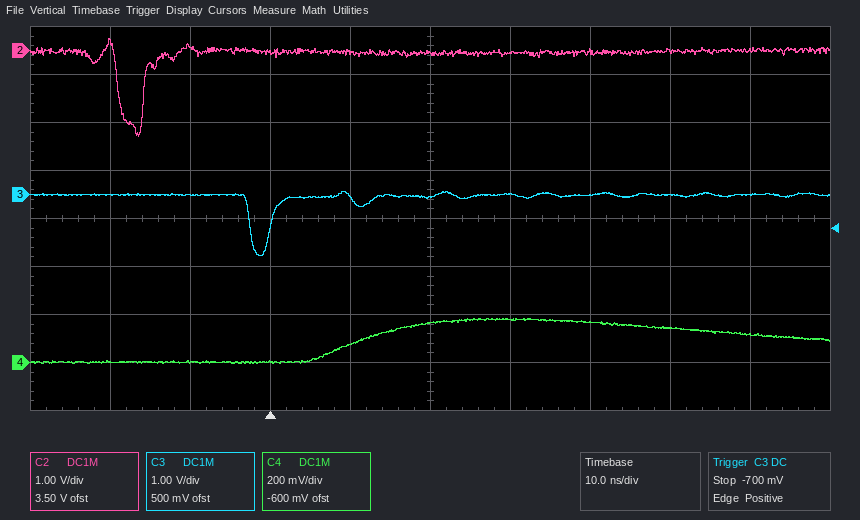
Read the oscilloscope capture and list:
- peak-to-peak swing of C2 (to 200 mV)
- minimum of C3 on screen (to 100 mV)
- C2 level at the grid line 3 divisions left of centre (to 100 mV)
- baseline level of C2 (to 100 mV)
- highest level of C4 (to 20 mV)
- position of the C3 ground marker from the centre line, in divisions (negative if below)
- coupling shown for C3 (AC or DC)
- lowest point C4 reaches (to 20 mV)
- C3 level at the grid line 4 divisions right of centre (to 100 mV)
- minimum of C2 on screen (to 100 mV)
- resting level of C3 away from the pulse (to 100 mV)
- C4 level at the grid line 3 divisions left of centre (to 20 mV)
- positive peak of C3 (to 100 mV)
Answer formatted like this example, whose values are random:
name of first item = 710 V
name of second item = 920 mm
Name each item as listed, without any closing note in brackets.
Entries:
peak-to-peak swing of C2 = 2.0 V
minimum of C3 on screen = -1.3 V
C2 level at the grid line 3 divisions left of centre = 100 mV
baseline level of C2 = 0.0 V
highest level of C4 = 180 mV
position of the C3 ground marker from the centre line, in divisions = +0.5 div
coupling shown for C3 = DC
lowest point C4 reaches = 0 mV
C3 level at the grid line 4 divisions right of centre = 0.0 V
minimum of C2 on screen = -1.8 V
resting level of C3 away from the pulse = 0.0 V
C4 level at the grid line 3 divisions left of centre = 0 mV
positive peak of C3 = 100 mV
